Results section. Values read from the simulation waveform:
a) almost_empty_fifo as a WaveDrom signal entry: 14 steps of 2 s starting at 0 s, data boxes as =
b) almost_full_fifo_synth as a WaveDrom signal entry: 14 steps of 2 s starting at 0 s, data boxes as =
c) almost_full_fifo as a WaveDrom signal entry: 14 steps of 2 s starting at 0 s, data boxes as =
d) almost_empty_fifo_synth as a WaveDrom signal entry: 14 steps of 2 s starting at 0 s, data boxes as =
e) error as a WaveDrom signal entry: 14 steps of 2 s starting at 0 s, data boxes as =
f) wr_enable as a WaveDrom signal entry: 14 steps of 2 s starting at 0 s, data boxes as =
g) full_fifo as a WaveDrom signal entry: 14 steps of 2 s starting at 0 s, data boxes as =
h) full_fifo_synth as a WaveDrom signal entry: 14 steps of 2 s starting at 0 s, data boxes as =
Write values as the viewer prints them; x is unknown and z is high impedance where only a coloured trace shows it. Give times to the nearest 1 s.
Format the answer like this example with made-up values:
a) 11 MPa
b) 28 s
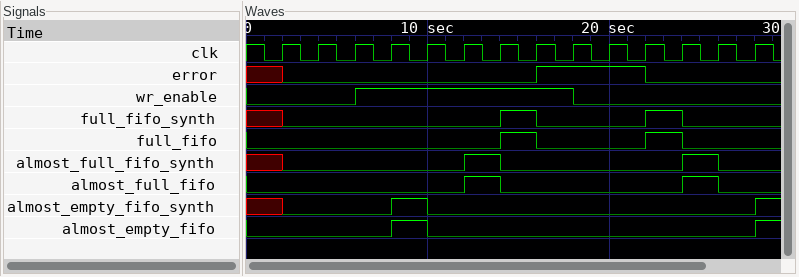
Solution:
a) {name: 'almost_empty_fifo', wave: '0...10........'}
b) {name: 'almost_full_fifo_synth', wave: 'x0....10....10'}
c) {name: 'almost_full_fifo', wave: '0.....10....10'}
d) {name: 'almost_empty_fifo_synth', wave: 'x0..10........'}
e) {name: 'error', wave: 'x0......1..0..'}
f) {name: 'wr_enable', wave: '0..1.....0....'}
g) {name: 'full_fifo', wave: '0......10..10.'}
h) {name: 'full_fifo_synth', wave: 'x0.....10..10.'}
